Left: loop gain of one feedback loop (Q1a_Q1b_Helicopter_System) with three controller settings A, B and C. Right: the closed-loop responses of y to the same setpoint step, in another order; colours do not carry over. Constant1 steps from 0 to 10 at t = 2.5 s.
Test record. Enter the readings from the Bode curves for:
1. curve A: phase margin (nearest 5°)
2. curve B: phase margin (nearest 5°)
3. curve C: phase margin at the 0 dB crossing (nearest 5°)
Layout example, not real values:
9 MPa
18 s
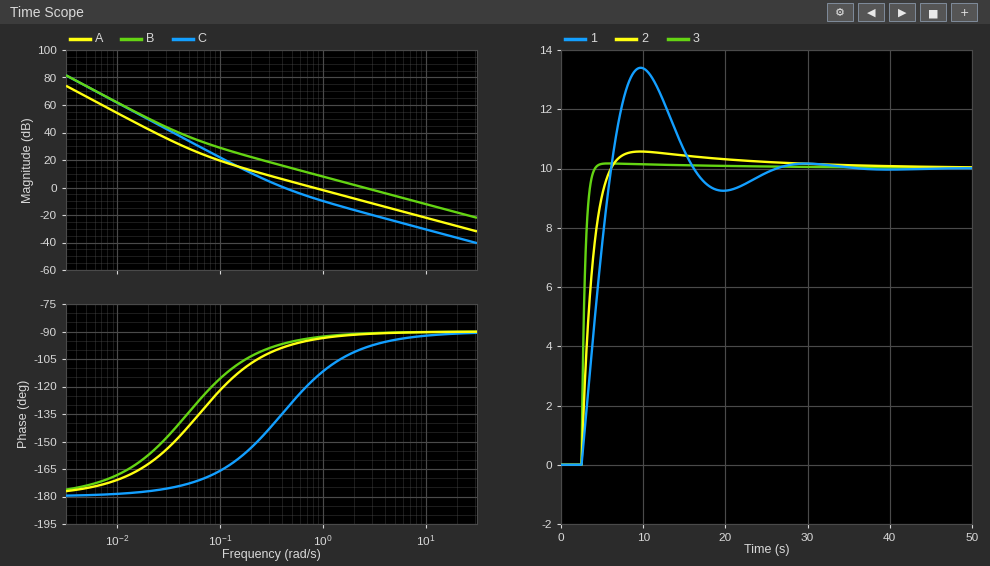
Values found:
85°
90°
45°
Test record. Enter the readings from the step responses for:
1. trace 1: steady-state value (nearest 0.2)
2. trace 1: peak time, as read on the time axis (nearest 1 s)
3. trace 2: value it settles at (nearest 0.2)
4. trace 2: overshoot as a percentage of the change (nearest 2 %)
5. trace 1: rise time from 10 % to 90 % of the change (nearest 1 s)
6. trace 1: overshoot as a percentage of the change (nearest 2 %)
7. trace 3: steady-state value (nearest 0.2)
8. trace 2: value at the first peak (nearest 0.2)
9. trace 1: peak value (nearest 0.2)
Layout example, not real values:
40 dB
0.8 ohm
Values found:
10.0
10 s
10.0
6 %
3 s
34 %
10.0
10.6
13.4
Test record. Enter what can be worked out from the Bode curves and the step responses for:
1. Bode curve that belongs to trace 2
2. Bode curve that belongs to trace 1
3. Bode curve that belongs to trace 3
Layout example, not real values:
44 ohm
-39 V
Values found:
A
C
B
